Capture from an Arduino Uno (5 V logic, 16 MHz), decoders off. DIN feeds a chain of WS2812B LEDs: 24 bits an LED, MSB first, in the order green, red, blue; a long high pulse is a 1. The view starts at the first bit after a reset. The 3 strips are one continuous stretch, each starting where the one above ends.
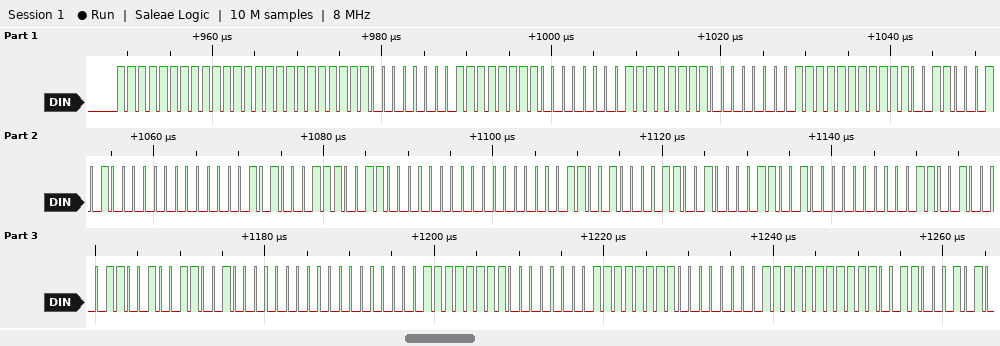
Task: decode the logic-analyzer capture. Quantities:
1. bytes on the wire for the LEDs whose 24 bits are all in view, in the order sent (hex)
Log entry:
FF FF FF 00 FF 00 FF 00 FF E6 28 00 28 E6 00 00 C8 64 32 00 64 32 64 00 00 FF 00 FF 00 FF
